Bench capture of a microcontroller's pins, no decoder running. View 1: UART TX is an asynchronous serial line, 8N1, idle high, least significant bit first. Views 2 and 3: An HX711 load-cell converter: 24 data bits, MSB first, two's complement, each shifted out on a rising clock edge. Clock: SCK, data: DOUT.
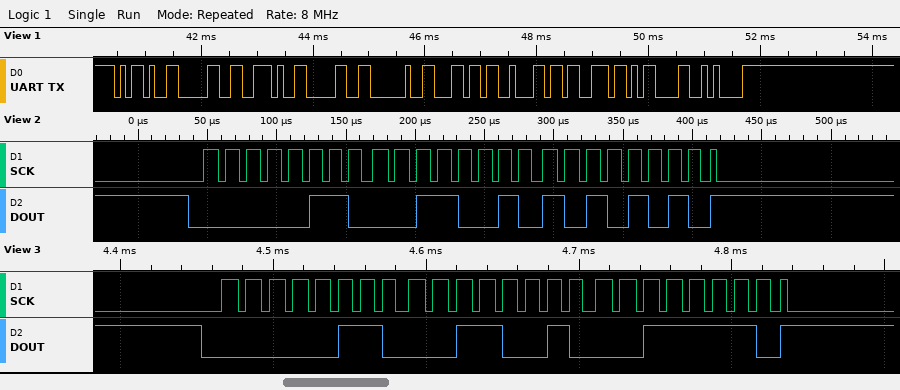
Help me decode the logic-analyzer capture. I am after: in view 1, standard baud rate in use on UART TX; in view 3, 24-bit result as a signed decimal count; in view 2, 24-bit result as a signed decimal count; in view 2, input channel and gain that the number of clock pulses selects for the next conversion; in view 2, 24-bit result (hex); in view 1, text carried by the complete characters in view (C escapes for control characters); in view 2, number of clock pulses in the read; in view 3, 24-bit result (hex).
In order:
9600 baud
406078
406186
channel A, gain 128
0x0632AA
"-0.0 lbs\r\n"
25
0x06323E
